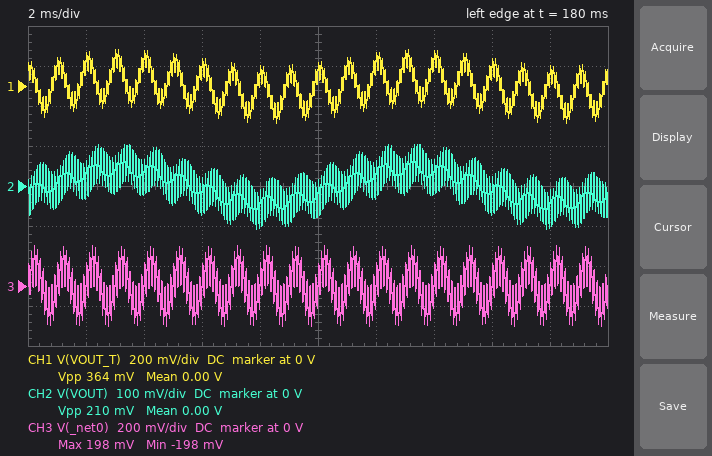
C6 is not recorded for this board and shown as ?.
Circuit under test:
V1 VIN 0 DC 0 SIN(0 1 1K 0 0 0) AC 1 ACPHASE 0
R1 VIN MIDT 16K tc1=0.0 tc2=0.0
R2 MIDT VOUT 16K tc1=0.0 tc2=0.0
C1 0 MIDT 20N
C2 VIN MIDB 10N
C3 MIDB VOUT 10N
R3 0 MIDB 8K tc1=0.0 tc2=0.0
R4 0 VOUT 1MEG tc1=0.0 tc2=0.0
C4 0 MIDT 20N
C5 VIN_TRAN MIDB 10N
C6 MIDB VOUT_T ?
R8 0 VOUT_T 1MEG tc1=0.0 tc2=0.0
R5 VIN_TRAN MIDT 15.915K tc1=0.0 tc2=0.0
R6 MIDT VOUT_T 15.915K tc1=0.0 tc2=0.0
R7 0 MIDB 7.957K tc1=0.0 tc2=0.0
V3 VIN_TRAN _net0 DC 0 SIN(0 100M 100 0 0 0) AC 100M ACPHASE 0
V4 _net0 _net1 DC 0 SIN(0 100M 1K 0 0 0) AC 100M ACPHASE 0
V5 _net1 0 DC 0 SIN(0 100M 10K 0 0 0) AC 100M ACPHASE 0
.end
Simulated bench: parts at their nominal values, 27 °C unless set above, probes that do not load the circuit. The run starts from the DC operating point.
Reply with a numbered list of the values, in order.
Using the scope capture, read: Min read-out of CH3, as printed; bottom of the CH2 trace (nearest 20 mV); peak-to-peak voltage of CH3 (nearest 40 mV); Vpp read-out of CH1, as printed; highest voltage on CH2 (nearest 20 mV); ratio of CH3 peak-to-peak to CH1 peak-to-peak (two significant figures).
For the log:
1. -198 mV
2. -100 mV
3. 400 mV
4. 364 mV
5. 100 mV
6. 1.1
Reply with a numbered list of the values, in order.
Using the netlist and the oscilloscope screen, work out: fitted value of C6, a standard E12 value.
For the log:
1. 27 nF
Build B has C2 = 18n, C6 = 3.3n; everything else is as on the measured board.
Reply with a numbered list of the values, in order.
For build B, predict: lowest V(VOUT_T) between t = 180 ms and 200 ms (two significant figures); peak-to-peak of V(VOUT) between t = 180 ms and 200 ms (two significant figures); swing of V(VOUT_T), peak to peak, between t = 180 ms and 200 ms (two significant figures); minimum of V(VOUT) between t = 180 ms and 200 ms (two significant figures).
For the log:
1. -160 mV
2. 340 mV
3. 320 mV
4. -170 mV
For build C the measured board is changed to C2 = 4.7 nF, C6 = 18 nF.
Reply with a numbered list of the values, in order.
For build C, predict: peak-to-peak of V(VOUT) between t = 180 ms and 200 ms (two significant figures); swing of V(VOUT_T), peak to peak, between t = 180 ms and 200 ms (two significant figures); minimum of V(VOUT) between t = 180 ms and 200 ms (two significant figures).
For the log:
1. 340 mV
2. 230 mV
3. -170 mV
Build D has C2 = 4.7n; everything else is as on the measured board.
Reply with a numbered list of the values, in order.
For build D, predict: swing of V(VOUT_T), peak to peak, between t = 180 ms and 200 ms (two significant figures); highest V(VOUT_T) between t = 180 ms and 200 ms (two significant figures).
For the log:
1. 250 mV
2. 120 mV
